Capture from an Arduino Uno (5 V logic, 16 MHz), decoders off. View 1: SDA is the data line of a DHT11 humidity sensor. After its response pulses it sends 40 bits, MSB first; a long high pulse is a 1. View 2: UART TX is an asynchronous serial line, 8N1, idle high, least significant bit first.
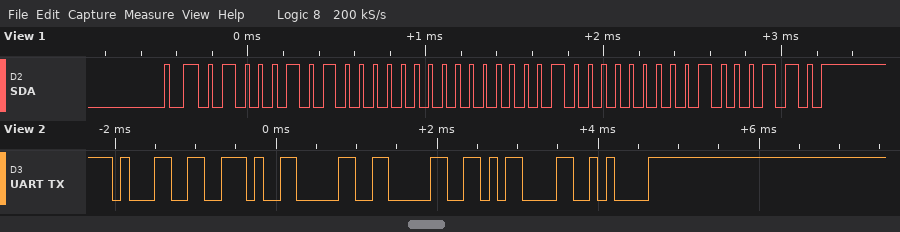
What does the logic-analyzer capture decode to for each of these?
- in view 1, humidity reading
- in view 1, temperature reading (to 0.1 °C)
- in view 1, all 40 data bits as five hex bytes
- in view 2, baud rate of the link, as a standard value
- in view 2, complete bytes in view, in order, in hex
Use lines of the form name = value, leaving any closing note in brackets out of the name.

in view 1, humidity reading = 69 %
in view 1, temperature reading = 1.0 °C
in view 1, all 40 data bits as five hex bytes = 45 00 01 00 46
in view 2, baud rate of the link, as a standard value = 9600 baud
in view 2, complete bytes in view, in order, in hex = 31 2E 30 30 0D 0A
